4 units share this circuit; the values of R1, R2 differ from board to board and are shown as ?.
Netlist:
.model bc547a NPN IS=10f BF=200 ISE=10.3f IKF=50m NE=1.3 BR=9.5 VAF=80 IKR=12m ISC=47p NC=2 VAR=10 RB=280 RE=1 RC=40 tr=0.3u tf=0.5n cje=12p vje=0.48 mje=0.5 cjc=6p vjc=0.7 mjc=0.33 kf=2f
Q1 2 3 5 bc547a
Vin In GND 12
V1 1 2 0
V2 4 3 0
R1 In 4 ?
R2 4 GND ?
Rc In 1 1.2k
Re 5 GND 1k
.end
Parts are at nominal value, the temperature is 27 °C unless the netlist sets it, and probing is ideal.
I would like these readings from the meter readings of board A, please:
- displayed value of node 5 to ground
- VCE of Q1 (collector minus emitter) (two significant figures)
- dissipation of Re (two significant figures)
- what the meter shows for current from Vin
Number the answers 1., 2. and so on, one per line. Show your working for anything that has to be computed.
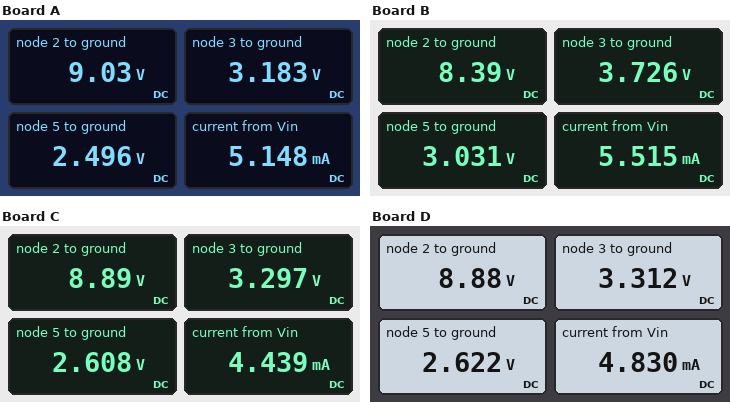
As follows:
1. 2.496 V
2. 9.03 V - 2.496 V = 6.5 V
3. (2.496 V)^2 / 1 kΩ = 6.2 mW
4. 5.148 mA
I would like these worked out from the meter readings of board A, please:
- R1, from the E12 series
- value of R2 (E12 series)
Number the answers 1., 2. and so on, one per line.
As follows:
1. 3.3 kΩ
2. 1.2 kΩ
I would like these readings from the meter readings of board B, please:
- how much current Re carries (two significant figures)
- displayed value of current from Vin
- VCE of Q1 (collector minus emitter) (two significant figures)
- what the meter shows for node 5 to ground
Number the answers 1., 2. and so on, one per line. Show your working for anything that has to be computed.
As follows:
1. (3.031 V) / 1 kΩ = 3.0 mA
2. 5.515 mA
3. 8.39 V - 3.031 V = 5.4 V
4. 3.031 V
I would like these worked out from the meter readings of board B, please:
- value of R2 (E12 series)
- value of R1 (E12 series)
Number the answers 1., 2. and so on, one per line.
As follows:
1. 1.5 kΩ
2. 3.3 kΩ
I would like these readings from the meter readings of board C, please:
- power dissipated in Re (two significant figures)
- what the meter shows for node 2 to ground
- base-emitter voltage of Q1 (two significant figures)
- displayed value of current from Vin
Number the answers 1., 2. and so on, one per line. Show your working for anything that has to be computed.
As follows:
1. (2.608 V)^2 / 1 kΩ = 6.8 mW
2. 8.89 V
3. 3.297 V - 2.608 V = 690 mV
4. 4.439 mA
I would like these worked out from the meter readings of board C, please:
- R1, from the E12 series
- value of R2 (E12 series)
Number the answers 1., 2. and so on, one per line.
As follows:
1. 4.7 kΩ
2. 1.8 kΩ
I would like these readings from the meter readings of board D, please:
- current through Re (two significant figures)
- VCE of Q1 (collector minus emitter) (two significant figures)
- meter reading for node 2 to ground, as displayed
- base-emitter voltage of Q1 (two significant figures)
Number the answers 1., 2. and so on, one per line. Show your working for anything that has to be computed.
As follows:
1. (2.622 V) / 1 kΩ = 2.6 mA
2. 8.88 V - 2.622 V = 6.3 V
3. 8.88 V
4. 3.312 V - 2.622 V = 690 mV
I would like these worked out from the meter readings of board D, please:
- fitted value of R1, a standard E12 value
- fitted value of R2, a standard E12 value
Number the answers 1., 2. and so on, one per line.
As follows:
1. 3.9 kΩ
2. 1.5 kΩ
